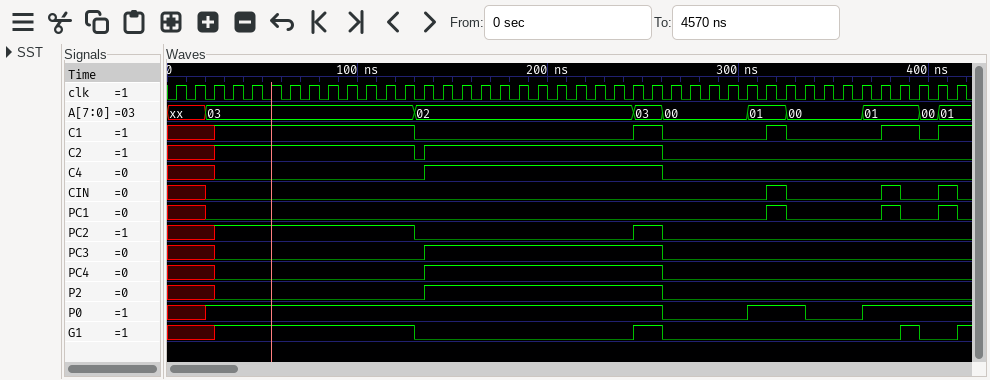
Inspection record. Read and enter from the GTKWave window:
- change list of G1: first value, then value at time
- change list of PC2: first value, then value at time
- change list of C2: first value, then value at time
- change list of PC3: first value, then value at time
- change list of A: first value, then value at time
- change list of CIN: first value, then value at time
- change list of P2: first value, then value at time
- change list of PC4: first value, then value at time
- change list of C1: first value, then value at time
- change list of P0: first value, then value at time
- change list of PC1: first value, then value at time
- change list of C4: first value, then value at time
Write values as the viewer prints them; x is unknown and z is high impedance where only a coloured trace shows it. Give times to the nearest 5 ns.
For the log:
x, 1 at 25 ns, 0 at 130 ns, 1 at 245 ns, 0 at 260 ns, 1 at 385 ns, 0 at 395 ns, 1 at 415 ns
x, 1 at 25 ns, 0 at 130 ns, 1 at 245 ns, 0 at 260 ns
x, 1 at 25 ns, 0 at 130 ns, 1 at 135 ns, 0 at 260 ns
x, 0 at 25 ns, 1 at 135 ns, 0 at 260 ns
xx, 03 at 20 ns, 02 at 130 ns, 03 at 245 ns, 00 at 260 ns, 01 at 305 ns, 00 at 325 ns, 01 at 365 ns, 00 at 395 ns, 01 at 405 ns
x, 0 at 20 ns, 1 at 315 ns, 0 at 325 ns, 1 at 375 ns, 0 at 385 ns, 1 at 405 ns, 0 at 415 ns
x, 0 at 25 ns, 1 at 135 ns, 0 at 260 ns
x, 0 at 25 ns, 1 at 135 ns, 0 at 260 ns
x, 1 at 25 ns, 0 at 130 ns, 1 at 245 ns, 0 at 260 ns, 1 at 315 ns, 0 at 325 ns, 1 at 375 ns, 0 at 395 ns, 1 at 405 ns
x, 1 at 20 ns, 0 at 260 ns, 1 at 305 ns, 0 at 335 ns, 1 at 365 ns
x, 0 at 20 ns, 1 at 315 ns, 0 at 325 ns, 1 at 375 ns, 0 at 385 ns, 1 at 405 ns, 0 at 415 ns
x, 0 at 25 ns, 1 at 135 ns, 0 at 260 ns
